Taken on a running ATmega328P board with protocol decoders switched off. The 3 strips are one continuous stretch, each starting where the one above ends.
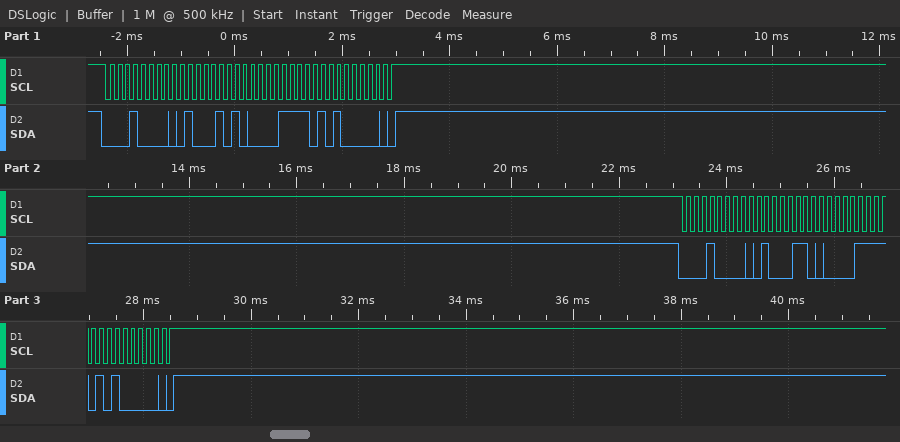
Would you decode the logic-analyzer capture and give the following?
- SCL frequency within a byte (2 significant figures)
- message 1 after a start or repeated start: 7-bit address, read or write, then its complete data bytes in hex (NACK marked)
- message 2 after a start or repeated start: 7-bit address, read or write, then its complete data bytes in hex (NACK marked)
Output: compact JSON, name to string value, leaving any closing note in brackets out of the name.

{"SCL frequency within a byte": "6.9 kHz", "message 1 after a start or repeated start: 7-bit address, read or write, then its complete data bytes in hex": "0x08 write: 45 0F A0", "message 2 after a start or repeated start: 7-bit address, read or write, then its complete data bytes in hex": "0x08 write: 46 0F A0"}
